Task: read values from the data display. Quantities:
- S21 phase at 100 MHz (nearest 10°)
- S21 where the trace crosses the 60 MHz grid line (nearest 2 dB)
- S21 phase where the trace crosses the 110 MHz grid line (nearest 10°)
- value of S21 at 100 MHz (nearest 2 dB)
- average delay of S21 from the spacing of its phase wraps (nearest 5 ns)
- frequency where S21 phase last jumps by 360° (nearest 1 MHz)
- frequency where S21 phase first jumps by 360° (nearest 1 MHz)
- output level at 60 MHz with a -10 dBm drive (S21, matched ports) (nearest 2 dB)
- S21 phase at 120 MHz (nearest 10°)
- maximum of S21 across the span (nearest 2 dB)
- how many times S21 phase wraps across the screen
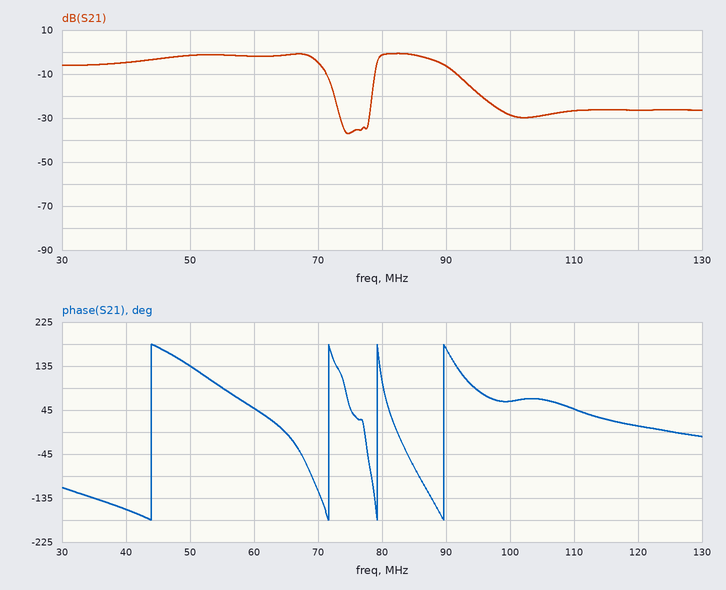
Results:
60°
-2 dB
50°
-28 dB
65 ns
90 MHz
44 MHz
-12 dBm
10°
0 dB
4
